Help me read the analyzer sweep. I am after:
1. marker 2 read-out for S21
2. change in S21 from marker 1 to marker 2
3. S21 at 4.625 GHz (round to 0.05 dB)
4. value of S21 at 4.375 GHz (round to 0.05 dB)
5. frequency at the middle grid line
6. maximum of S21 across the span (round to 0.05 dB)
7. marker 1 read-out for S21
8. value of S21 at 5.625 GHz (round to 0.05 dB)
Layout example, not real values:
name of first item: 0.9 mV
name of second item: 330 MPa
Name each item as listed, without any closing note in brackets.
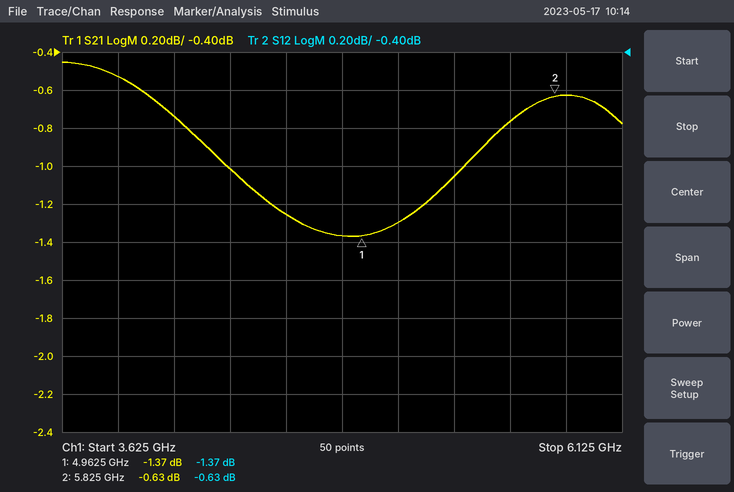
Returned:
marker 2 read-out for S21: -0.63 dB
change in S21 from marker 1 to marker 2: 0.74 dB
S21 at 4.625 GHz: -1.25 dB
value of S21 at 4.375 GHz: -1.00 dB
frequency at the middle grid line: 4.875 GHz
maximum of S21 across the span: -0.45 dB
marker 1 read-out for S21: -1.37 dB
value of S21 at 5.625 GHz: -0.75 dB
